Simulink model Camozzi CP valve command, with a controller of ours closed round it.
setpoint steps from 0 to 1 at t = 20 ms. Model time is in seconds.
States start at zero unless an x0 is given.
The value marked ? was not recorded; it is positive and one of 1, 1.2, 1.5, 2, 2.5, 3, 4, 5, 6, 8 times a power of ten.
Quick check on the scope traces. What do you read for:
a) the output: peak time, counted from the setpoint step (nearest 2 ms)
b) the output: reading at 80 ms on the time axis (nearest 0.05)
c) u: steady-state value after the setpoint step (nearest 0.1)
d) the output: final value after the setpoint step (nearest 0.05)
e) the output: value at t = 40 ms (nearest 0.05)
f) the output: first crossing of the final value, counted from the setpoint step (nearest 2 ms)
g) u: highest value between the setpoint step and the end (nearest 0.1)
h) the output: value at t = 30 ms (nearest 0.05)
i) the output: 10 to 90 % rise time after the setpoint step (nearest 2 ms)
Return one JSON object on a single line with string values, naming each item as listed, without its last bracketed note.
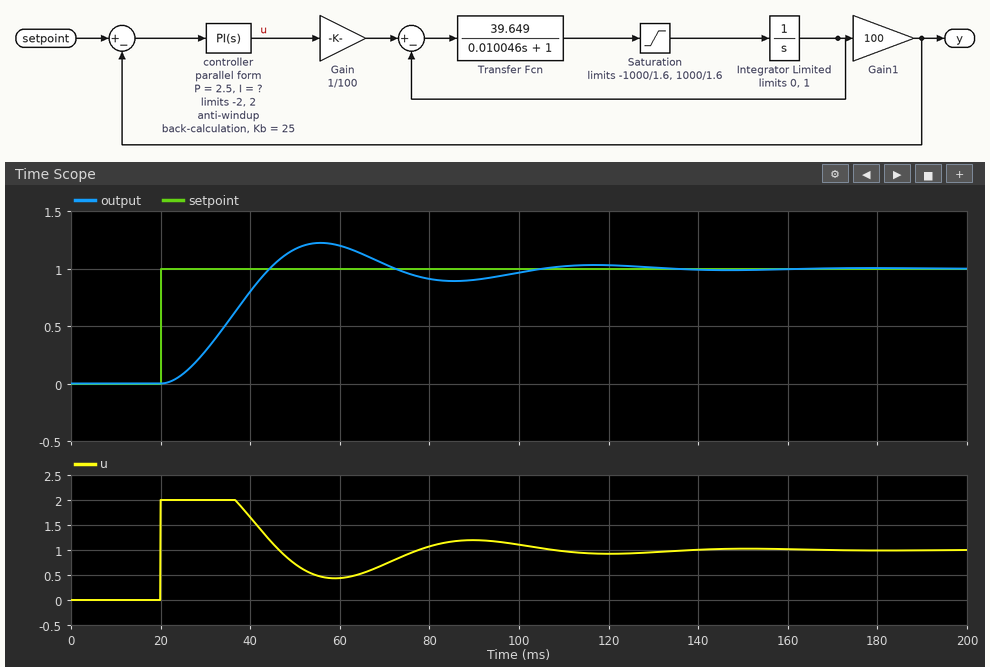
{"the output: peak time, counted from the setpoint step": "36 ms", "the output: reading at 80 ms on the time axis": "0.90", "u: steady-state value after the setpoint step": "1.0", "the output: final value after the setpoint step": "1.00", "the output: value at t = 40 ms": "0.80", "the output: first crossing of the final value, counted from the setpoint step": "24 ms", "u: highest value between the setpoint step and the end": "2.0", "the output: value at t = 30 ms": "0.30", "the output: 10 to 90 % rise time after the setpoint step": "16 ms"}
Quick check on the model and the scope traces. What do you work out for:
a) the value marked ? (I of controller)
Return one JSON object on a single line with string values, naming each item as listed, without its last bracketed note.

{"the value marked ?": "100"}
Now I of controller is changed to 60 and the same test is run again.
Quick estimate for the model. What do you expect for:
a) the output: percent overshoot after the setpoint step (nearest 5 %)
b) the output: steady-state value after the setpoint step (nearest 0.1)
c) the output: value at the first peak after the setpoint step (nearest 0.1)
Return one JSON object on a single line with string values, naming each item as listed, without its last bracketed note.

{"the output: percent overshoot after the setpoint step": "10 %", "the output: steady-state value after the setpoint step": "1.0", "the output: value at the first peak after the setpoint step": "1.1"}
